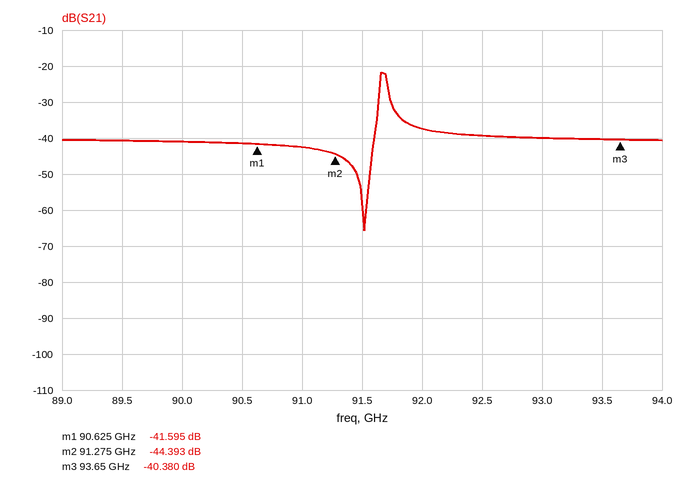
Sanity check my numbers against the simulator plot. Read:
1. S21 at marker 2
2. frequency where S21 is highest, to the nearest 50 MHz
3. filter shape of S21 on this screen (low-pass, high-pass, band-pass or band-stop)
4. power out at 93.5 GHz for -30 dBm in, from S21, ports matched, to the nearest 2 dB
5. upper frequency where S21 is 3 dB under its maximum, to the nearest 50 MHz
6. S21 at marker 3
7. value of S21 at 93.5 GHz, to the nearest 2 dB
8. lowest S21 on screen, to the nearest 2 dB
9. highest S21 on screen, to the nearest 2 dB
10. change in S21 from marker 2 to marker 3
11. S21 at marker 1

-44.393 dB
91.65 GHz
band-pass
-70 dBm
91.70 GHz
-40.380 dB
-40 dB
-66 dB
-22 dB
4.013 dB
-41.595 dB
